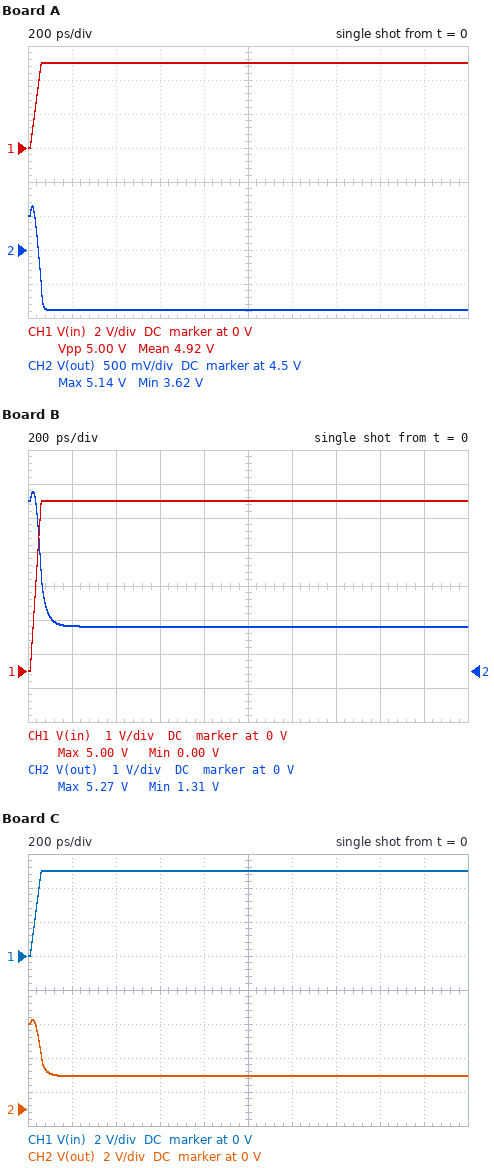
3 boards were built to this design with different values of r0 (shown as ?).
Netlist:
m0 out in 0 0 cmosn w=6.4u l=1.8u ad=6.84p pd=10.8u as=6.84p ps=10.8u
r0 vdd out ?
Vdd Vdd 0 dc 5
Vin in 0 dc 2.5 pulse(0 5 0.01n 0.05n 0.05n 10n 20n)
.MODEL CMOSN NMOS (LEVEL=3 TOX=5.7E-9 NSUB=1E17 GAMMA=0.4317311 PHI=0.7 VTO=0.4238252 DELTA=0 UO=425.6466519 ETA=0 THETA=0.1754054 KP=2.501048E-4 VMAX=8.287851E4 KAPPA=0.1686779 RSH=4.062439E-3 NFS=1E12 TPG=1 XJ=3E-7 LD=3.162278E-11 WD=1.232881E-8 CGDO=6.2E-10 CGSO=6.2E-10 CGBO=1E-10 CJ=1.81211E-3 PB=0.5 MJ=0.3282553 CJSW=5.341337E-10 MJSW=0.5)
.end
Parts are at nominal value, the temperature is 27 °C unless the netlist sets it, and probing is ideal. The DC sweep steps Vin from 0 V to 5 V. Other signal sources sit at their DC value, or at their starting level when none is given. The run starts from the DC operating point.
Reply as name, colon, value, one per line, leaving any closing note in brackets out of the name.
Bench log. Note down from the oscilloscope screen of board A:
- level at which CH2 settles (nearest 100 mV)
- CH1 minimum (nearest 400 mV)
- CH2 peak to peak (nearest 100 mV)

level at which CH2 settles: 3.6 V
CH1 minimum: 0 V
CH2 peak to peak: 1.5 V
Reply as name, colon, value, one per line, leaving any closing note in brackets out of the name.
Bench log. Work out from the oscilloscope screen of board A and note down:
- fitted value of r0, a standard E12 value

fitted value of r0, a standard E12 value: 470 Ω
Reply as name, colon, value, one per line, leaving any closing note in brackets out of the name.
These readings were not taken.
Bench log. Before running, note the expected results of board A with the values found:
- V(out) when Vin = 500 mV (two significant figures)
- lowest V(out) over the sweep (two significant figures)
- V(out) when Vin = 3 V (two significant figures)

V(out) when Vin = 500 mV: 5.0 V
lowest V(out) over the sweep: 3.6 V
V(out) when Vin = 3 V: 4.4 V
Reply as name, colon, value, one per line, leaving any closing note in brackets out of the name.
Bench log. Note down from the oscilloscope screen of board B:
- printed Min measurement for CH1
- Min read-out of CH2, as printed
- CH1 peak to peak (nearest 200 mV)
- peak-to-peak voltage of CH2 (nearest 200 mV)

printed Min measurement for CH1: 0.00 V
Min read-out of CH2, as printed: 1.31 V
CH1 peak to peak: 5.0 V
peak-to-peak voltage of CH2: 4.0 V
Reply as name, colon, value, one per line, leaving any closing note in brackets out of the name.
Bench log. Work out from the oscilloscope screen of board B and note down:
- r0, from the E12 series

r0, from the E12 series: 1.8 kΩ
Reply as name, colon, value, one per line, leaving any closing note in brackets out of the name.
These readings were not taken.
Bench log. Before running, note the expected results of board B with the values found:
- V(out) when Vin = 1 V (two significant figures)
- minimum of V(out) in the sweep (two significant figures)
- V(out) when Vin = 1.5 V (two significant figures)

V(out) when Vin = 1 V: 4.8 V
minimum of V(out) in the sweep: 1.3 V
V(out) when Vin = 1.5 V: 4.4 V
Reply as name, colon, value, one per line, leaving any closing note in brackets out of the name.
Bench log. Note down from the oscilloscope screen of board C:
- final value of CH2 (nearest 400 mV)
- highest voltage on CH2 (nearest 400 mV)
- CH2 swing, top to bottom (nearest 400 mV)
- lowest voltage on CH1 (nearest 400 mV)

final value of CH2: 2.0 V
highest voltage on CH2: 5.2 V
CH2 swing, top to bottom: 3.2 V
lowest voltage on CH1: 0 V
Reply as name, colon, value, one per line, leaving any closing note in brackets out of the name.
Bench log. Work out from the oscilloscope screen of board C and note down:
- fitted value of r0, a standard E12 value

fitted value of r0, a standard E12 value: 1.2 kΩ
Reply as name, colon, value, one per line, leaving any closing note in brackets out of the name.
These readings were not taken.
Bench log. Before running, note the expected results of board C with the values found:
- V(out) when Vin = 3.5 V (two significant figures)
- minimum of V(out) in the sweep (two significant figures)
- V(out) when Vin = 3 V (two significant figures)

V(out) when Vin = 3.5 V: 3.0 V
minimum of V(out) in the sweep: 1.9 V
V(out) when Vin = 3 V: 3.4 V
